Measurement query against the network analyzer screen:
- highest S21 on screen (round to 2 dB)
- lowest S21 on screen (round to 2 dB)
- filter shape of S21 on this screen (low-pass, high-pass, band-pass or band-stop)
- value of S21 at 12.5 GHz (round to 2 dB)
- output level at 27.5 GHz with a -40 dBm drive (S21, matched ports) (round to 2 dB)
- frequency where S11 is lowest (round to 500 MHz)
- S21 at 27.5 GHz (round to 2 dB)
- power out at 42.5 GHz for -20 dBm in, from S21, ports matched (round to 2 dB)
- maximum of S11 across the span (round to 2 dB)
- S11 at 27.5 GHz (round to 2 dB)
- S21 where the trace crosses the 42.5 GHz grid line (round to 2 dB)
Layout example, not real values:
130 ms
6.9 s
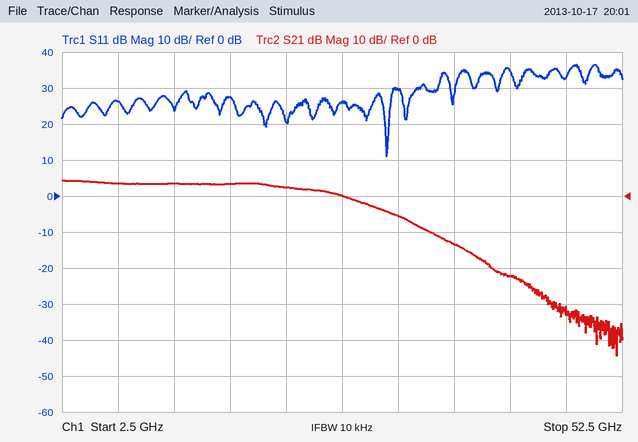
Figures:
4 dB
-44 dB
low-pass
4 dB
-40 dBm
31.5 GHz
0 dB
-42 dBm
36 dB
26 dB
-22 dB
